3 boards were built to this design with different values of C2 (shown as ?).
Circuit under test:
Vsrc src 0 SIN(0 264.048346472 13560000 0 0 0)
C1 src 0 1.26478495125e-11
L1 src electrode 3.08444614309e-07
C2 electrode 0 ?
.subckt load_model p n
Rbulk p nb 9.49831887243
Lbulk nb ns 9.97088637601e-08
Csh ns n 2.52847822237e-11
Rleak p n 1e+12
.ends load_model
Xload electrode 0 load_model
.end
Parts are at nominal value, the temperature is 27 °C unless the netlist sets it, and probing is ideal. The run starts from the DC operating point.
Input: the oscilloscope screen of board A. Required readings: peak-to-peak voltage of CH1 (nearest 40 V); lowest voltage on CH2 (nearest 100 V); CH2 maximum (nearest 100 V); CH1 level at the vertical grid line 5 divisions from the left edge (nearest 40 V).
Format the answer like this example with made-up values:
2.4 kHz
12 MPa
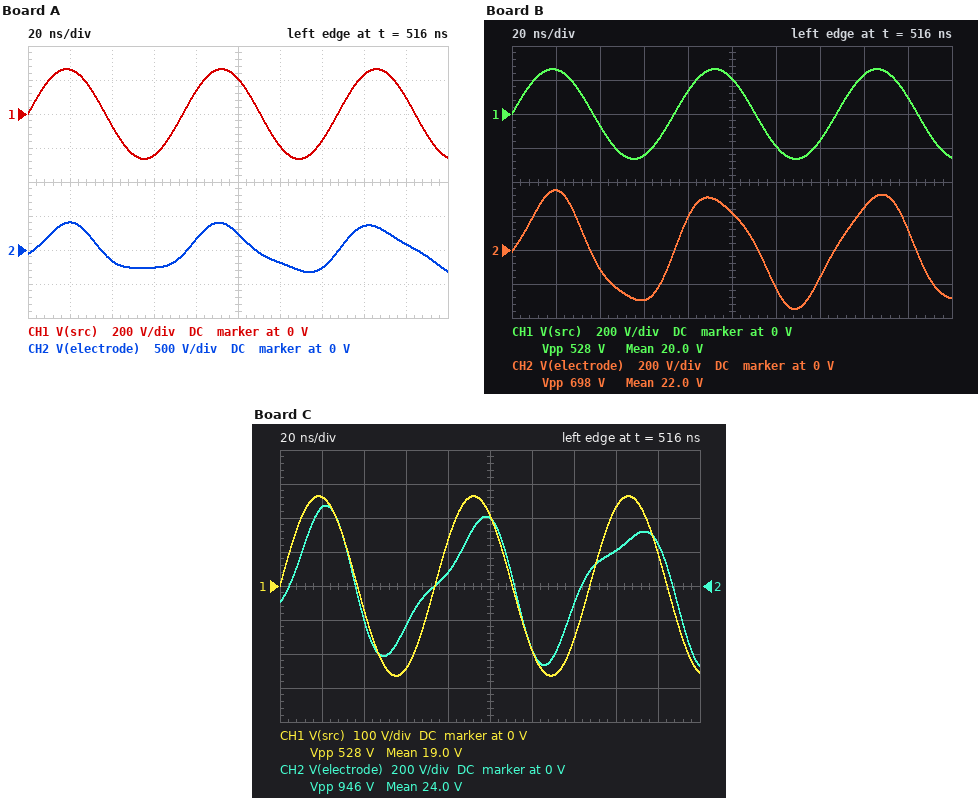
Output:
520 V
-300 V
400 V
200 V
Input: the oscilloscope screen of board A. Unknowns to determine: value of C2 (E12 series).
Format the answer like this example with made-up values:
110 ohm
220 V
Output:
68 pF
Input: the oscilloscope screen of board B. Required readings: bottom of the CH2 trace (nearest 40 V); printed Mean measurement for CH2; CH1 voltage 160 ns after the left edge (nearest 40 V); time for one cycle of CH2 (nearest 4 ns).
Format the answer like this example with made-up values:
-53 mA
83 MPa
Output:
-360 V
22.0 V
240 V
72 ns
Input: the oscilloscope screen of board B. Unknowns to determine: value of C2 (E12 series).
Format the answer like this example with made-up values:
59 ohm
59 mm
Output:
47 pF
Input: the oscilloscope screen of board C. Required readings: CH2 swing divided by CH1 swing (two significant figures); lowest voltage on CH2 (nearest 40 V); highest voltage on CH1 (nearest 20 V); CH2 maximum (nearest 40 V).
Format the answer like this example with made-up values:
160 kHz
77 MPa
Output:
1.8
-480 V
260 V
480 V
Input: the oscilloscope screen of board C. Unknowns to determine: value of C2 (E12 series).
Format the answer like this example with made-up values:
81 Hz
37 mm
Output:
100 pF
